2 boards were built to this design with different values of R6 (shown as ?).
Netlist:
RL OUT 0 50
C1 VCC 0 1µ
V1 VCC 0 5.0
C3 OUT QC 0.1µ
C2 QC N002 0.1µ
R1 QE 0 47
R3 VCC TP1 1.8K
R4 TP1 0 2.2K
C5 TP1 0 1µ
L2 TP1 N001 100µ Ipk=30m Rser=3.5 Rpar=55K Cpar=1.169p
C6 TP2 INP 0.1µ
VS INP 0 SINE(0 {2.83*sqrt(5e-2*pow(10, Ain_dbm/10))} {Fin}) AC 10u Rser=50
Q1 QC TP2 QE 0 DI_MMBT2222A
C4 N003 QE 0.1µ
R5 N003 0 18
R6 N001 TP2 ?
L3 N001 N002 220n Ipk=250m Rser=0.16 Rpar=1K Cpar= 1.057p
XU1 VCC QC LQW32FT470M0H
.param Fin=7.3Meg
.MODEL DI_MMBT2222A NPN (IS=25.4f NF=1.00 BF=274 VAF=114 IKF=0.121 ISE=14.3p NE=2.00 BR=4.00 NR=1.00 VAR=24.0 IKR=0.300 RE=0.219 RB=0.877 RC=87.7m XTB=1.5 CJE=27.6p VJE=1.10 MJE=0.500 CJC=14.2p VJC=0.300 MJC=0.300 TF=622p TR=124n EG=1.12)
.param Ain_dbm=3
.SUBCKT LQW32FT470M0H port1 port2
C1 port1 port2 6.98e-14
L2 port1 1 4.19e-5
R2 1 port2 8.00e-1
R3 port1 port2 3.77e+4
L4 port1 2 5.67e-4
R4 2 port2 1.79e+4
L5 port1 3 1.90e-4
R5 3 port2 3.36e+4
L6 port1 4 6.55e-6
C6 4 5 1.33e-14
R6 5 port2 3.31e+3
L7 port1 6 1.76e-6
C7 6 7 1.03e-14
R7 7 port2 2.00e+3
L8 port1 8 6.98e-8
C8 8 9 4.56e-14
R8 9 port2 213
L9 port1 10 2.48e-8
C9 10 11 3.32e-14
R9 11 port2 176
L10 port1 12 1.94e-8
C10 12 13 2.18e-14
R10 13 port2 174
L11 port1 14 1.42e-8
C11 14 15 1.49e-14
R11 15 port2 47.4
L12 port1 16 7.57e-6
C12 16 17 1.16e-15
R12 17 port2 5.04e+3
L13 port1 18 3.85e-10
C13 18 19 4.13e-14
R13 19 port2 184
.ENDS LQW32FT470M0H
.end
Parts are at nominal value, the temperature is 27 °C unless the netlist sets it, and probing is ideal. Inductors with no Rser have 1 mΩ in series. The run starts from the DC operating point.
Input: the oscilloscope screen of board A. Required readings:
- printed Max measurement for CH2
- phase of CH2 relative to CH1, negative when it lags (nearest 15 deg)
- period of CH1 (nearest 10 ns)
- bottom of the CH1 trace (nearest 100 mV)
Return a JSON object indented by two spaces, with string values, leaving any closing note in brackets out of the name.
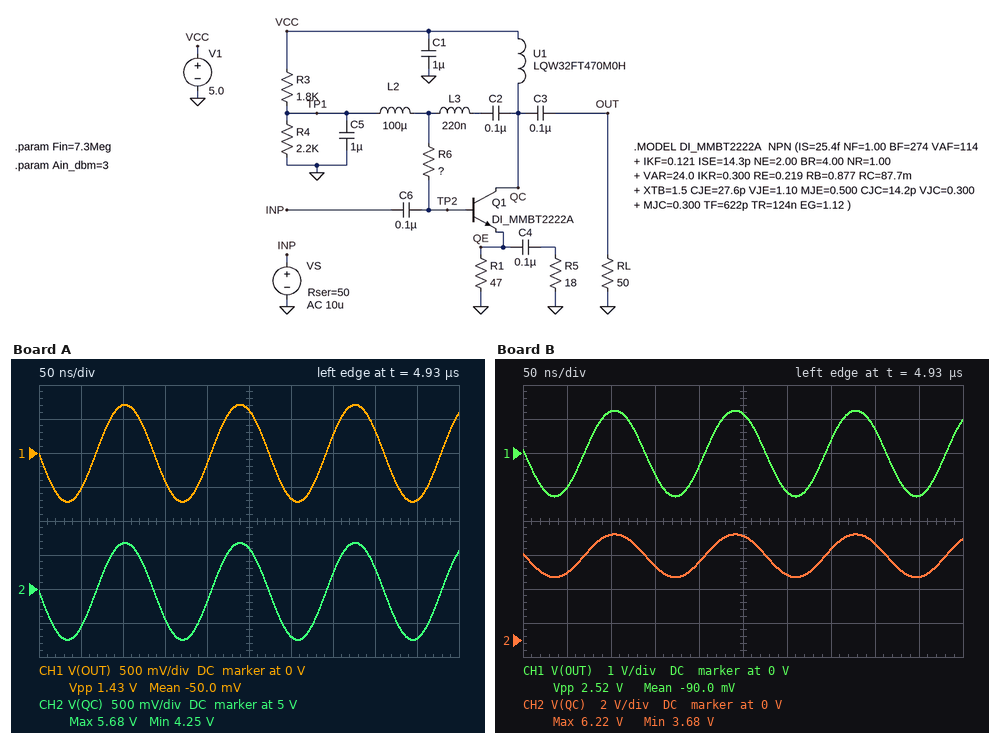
{
  "printed Max measurement for CH2": "5.68 V",
  "phase of CH2 relative to CH1, negative when it lags": "0 deg",
  "period of CH1": "140 ns",
  "bottom of the CH1 trace": "-700 mV"
}
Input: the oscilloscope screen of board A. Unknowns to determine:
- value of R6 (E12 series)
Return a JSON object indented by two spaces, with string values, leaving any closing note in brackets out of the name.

{
  "value of R6": "100 Ω"
}
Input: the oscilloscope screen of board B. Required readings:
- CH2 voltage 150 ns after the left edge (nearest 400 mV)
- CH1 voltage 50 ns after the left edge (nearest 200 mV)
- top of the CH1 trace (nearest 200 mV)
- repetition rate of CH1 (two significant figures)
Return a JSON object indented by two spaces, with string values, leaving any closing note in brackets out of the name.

{
  "CH2 voltage 150 ns after the left edge": "4.4 V",
  "CH1 voltage 50 ns after the left edge": "-1.0 V",
  "top of the CH1 trace": "1.2 V",
  "repetition rate of CH1": "7.3 MHz"
}
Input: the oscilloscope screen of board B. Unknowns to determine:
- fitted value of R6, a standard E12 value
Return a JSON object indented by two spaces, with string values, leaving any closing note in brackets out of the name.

{
  "fitted value of R6, a standard E12 value": "220 Ω"
}
